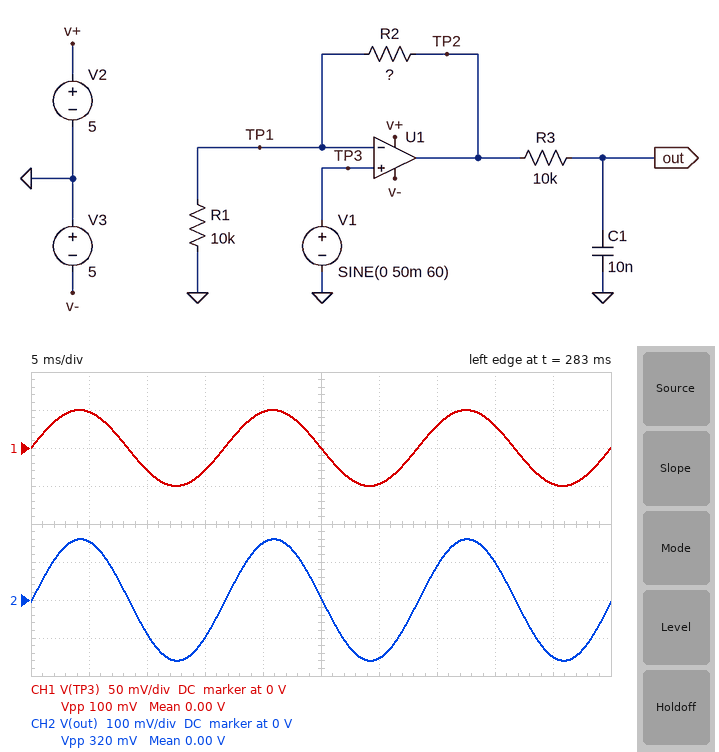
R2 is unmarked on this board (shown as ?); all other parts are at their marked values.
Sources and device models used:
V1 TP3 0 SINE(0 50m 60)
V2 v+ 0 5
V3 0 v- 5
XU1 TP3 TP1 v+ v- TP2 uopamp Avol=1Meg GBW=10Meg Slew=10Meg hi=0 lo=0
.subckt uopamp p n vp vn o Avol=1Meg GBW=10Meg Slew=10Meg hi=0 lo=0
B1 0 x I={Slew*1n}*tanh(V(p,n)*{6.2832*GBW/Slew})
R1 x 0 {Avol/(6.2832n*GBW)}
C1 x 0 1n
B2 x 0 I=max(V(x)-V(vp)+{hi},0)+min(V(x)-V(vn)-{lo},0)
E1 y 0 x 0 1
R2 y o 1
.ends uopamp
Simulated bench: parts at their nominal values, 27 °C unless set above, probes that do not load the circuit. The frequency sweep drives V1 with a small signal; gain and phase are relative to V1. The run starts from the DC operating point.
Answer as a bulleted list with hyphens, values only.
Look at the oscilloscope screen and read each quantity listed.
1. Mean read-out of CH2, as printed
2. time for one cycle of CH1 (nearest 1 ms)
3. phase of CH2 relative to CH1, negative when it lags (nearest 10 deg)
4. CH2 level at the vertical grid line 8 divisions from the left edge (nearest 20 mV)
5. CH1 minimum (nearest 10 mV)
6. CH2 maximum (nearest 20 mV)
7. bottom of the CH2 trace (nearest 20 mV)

- 0.00 V
- 17 ms
- 0 deg
- 100 mV
- -50 mV
- 160 mV
- -160 mV
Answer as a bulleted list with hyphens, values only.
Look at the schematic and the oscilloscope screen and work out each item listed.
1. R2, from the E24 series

- 22 kΩ
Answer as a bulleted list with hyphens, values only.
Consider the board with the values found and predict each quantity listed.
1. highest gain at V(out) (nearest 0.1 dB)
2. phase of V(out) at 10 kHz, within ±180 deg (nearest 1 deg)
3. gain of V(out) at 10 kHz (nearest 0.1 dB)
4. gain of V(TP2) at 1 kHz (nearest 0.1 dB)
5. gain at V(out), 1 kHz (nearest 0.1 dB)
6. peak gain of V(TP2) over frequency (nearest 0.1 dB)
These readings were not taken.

- 10.1 dB
- -81 deg
- -6.0 dB
- 10.1 dB
- 8.7 dB
- 10.1 dB
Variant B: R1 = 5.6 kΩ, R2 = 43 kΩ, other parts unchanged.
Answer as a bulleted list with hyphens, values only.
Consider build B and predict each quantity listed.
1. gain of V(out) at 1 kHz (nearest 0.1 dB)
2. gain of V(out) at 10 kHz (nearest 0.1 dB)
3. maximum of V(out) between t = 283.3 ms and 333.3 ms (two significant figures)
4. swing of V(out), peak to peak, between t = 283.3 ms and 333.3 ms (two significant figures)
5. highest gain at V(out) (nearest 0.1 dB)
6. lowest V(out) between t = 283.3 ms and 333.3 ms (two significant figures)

- 17.3 dB
- 2.7 dB
- 430 mV
- 870 mV
- 18.8 dB
- -430 mV
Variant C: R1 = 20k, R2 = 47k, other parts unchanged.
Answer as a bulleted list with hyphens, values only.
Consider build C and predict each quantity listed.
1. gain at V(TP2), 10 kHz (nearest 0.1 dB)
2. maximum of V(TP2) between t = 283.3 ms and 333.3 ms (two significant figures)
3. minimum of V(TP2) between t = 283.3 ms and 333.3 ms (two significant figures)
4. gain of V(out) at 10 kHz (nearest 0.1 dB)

- 10.5 dB
- 170 mV
- -170 mV
- -5.6 dB
